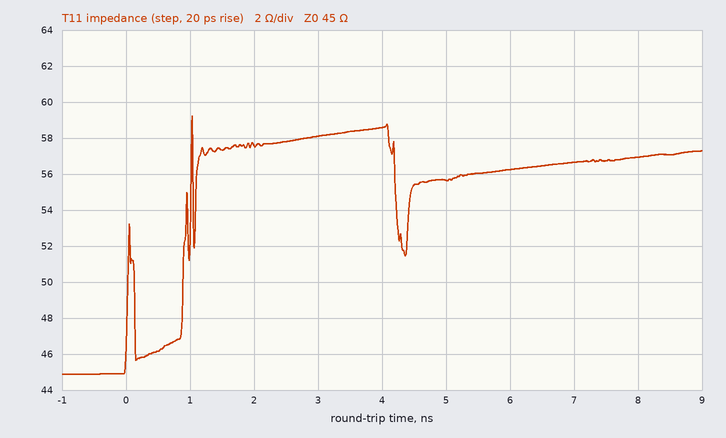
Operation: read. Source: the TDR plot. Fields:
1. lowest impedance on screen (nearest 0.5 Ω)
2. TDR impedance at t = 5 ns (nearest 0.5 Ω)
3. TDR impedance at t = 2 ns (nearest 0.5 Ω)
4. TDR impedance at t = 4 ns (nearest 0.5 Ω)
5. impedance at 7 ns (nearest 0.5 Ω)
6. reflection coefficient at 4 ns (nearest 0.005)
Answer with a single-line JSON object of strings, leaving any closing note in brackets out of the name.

{"lowest impedance on screen": "45.0 Ω", "TDR impedance at t = 5 ns": "55.5 Ω", "TDR impedance at t = 2 ns": "57.5 Ω", "TDR impedance at t = 4 ns": "58.5 Ω", "impedance at 7 ns": "56.5 Ω", "reflection coefficient at 4 ns": "+0.130"}
